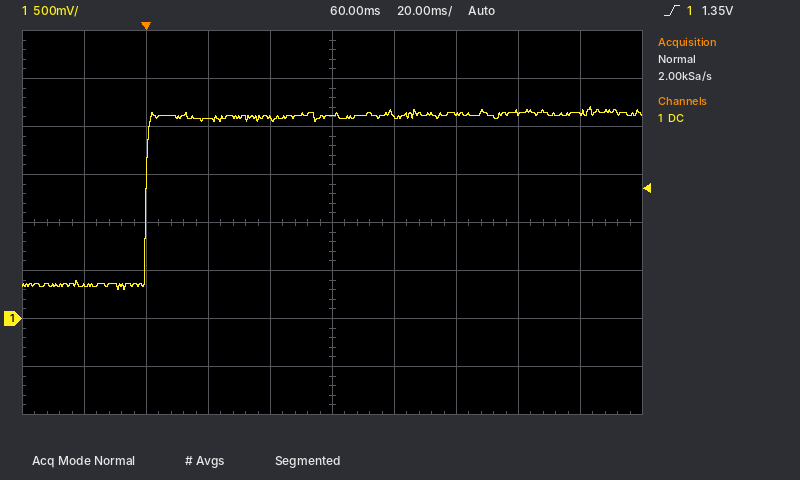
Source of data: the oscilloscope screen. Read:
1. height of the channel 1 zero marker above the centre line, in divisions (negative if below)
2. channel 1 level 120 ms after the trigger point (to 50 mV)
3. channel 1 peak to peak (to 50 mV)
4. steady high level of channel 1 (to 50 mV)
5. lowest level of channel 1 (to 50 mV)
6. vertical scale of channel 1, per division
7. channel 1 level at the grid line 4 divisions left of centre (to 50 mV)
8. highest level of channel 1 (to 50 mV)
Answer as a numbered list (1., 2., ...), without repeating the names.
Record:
1. -2.0 div
2. 2.15 V
3. 1.90 V
4. 2.10 V
5. 300 mV
6. 500 mV
7. 350 mV
8. 2.20 V
